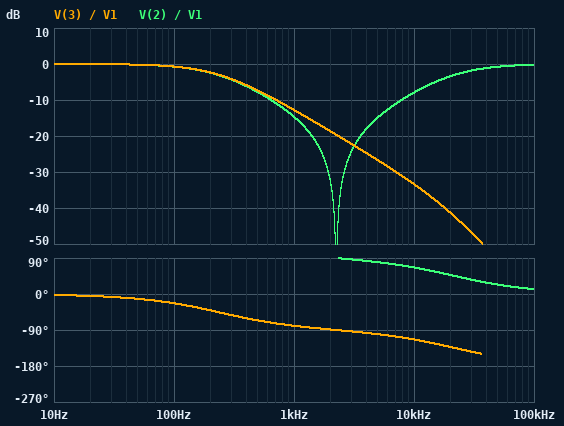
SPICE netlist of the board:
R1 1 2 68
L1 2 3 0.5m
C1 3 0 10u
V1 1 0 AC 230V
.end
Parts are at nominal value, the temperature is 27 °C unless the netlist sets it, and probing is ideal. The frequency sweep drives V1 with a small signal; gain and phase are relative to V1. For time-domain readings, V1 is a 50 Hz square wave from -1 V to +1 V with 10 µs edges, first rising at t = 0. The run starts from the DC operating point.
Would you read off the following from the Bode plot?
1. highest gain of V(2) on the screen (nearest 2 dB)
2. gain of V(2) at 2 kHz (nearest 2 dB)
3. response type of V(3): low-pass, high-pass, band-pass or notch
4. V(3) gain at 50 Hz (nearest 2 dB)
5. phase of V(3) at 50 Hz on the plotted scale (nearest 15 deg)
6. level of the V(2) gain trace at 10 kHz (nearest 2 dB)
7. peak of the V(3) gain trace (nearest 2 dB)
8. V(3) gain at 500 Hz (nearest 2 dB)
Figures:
0 dB
-32 dB
low-pass
0 dB
-15 deg
-8 dB
0 dB
-8 dB
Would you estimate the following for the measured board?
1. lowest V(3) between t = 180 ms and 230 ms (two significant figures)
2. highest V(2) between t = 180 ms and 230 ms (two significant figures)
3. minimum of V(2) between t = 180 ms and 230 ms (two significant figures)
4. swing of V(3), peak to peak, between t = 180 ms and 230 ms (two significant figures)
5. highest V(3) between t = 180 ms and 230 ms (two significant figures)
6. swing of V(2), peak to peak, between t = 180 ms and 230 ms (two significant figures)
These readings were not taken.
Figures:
-1.0 V
1.0 V
-1.0 V
2.0 V
1.0 V
2.0 V
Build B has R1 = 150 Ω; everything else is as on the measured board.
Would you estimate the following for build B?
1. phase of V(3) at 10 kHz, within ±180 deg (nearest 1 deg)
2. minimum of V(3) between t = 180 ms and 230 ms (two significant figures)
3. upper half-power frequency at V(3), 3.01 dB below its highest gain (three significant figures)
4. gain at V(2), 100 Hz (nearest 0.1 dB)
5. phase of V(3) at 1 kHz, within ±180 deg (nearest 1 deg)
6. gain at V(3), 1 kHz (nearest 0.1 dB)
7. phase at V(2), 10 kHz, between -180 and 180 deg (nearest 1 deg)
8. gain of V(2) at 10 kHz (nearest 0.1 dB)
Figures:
-101 deg
-1.0 V
106 Hz
-2.8 dB
-85 deg
-19.5 dB
79 deg
-14.2 dB
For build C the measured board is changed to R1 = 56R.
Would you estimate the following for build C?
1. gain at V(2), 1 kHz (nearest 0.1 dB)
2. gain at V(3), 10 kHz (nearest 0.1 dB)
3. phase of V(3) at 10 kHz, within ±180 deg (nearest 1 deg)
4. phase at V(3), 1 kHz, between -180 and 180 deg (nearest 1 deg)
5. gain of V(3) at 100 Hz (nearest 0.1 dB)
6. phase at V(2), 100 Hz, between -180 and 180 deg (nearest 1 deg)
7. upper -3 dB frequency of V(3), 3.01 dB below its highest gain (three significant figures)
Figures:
-13.1 dB
-32.0 dB
-118 deg
-77 deg
-0.5 dB
-19 deg
289 Hz
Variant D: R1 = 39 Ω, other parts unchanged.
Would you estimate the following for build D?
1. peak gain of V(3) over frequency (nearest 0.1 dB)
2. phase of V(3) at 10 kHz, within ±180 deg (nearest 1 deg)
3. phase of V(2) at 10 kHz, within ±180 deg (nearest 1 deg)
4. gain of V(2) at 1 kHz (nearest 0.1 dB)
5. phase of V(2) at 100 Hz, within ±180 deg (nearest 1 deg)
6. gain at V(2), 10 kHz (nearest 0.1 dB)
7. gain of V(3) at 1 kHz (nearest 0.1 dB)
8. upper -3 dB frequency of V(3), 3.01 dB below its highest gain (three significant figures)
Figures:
0 dB
-127 deg
53 deg
-10.1 dB
-14 deg
-4.3 dB
-8.2 dB
422 Hz
